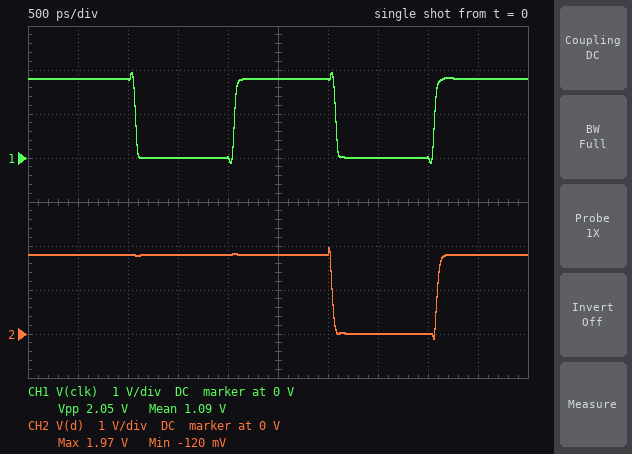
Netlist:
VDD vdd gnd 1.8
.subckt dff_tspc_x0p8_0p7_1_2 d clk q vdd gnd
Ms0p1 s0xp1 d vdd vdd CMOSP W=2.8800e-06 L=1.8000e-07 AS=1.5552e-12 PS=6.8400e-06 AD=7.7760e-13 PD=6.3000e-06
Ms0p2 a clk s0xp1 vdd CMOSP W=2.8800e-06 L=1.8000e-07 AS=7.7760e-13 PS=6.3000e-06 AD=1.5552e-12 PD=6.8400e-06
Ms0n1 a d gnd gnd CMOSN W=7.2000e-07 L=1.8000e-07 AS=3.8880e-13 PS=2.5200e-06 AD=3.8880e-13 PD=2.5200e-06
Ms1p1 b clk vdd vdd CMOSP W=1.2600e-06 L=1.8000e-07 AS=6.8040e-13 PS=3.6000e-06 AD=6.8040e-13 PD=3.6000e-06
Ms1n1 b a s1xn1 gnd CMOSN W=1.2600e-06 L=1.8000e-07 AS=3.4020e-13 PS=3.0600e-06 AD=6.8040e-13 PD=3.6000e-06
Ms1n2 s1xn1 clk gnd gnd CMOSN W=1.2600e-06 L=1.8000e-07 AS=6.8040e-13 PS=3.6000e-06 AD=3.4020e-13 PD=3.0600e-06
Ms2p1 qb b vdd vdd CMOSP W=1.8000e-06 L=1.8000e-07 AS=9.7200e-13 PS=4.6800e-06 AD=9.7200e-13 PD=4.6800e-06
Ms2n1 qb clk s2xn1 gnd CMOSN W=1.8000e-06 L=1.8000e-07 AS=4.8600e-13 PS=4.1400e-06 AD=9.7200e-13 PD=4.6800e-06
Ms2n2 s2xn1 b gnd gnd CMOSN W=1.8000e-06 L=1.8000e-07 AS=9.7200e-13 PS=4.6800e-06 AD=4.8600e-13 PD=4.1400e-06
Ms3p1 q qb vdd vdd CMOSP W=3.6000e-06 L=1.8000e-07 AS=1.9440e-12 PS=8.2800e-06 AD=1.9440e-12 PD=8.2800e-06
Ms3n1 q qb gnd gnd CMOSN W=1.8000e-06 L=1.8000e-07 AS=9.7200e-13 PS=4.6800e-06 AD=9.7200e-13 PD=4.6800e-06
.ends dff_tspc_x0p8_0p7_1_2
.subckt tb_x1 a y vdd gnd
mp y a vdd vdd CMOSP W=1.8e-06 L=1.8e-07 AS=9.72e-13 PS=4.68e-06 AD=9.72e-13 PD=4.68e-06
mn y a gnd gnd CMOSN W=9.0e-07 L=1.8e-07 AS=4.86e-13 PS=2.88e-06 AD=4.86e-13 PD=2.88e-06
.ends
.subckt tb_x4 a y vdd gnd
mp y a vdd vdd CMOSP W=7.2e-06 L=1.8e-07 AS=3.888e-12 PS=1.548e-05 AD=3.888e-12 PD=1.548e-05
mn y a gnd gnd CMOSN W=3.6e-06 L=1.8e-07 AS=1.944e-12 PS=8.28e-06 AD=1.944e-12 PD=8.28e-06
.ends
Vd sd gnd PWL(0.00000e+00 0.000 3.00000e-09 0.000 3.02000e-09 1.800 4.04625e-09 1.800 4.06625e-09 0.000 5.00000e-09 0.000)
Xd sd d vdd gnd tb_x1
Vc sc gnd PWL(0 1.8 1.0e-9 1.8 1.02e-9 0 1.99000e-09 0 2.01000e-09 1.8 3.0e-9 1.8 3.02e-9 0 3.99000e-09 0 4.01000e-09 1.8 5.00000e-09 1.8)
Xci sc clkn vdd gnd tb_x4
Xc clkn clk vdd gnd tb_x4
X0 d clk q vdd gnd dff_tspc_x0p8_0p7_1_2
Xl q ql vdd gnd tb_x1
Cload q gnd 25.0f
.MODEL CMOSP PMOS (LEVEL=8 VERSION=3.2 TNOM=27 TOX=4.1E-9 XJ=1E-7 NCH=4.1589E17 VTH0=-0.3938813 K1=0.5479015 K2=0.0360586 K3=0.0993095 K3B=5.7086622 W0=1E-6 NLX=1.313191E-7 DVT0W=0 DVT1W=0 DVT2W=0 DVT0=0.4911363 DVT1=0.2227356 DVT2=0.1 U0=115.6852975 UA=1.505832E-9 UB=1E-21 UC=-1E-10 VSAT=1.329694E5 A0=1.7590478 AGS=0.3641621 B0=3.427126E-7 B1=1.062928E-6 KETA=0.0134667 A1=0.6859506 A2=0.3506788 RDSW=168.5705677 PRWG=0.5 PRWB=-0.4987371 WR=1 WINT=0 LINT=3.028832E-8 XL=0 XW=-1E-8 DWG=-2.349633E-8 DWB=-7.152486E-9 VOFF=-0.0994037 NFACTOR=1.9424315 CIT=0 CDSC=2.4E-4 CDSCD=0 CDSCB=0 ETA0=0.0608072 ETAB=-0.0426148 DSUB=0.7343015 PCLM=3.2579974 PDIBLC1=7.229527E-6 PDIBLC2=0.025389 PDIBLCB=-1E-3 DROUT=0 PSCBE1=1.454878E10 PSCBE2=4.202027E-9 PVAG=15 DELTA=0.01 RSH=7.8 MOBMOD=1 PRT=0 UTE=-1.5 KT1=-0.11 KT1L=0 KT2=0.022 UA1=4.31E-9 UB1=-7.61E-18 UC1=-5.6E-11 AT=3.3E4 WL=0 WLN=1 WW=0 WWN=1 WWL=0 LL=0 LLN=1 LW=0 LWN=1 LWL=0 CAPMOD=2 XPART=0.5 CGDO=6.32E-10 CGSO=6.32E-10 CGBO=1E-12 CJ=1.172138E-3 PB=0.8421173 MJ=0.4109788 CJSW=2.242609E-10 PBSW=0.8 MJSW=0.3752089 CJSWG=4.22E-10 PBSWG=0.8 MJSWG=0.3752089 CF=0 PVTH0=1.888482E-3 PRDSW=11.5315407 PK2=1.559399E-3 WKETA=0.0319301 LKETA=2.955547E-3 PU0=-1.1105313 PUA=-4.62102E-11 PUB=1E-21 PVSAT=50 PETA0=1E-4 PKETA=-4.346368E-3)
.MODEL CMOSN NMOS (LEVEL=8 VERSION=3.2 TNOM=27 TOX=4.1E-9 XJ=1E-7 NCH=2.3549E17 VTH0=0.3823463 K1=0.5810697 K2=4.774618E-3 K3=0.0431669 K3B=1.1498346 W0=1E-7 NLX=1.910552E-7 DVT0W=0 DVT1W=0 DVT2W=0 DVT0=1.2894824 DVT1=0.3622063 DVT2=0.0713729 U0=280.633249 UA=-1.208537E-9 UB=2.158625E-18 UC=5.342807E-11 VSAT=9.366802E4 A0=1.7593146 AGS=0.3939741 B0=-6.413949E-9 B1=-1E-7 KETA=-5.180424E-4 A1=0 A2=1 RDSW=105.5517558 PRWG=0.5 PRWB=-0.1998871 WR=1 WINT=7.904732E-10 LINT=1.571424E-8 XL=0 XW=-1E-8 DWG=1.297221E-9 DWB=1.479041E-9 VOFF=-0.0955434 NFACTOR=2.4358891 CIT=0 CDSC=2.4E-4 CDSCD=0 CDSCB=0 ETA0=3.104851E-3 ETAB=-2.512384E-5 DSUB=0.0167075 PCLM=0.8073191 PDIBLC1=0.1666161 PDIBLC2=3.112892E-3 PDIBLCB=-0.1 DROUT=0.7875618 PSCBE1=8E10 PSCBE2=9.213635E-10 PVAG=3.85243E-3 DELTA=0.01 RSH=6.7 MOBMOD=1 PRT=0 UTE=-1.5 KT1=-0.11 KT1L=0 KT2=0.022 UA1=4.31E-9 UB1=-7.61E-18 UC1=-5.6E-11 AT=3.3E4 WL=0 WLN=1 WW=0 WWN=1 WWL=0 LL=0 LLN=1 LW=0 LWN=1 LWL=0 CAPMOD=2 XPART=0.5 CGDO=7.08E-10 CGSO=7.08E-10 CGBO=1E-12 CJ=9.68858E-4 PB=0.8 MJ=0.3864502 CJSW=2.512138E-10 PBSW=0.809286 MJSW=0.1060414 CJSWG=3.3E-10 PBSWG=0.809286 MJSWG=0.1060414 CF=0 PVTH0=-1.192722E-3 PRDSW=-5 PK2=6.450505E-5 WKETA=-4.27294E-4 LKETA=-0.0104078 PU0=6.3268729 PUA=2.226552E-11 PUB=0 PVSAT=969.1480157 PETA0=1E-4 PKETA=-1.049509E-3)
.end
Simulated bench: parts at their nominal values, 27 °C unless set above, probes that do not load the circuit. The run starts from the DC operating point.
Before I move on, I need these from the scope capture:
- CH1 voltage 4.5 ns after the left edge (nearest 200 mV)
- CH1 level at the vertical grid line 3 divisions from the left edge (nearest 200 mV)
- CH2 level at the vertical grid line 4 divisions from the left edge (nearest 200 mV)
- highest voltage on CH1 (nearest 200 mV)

1.8 V
0 V
1.8 V
2.0 V
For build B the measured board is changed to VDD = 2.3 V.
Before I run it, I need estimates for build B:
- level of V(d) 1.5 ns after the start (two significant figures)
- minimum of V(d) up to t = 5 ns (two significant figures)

2.3 V
-63 mV
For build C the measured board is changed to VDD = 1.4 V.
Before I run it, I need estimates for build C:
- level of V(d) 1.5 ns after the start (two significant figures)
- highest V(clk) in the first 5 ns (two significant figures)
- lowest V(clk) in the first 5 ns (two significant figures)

1.4 V
1.5 V
-160 mV
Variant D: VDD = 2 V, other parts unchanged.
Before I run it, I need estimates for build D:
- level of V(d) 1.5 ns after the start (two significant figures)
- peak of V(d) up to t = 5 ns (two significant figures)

2.0 V
2.2 V
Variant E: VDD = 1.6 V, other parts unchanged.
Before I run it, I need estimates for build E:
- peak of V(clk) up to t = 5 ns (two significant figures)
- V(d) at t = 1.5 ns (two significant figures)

1.7 V
1.6 V
